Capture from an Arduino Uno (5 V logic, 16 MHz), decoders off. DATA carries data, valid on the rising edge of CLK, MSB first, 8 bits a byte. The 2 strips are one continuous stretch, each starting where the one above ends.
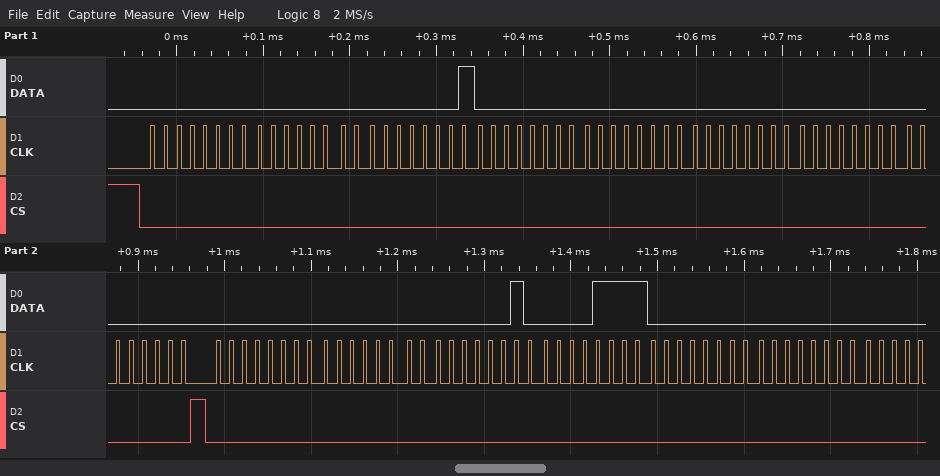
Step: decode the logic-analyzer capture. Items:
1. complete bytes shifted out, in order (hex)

00 00 01 00 00 00 00 00 00 00 02 0F 00 00
